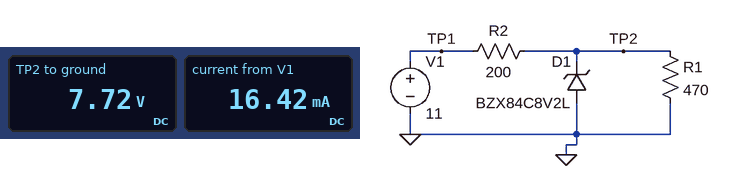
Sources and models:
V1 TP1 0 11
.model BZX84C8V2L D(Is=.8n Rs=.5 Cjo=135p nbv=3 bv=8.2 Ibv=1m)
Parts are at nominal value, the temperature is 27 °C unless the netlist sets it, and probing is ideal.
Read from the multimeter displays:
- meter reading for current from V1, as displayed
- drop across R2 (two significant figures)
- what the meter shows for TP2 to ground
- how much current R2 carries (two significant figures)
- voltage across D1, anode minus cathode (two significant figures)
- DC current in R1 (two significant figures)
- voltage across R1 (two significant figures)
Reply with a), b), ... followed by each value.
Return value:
a) 16.42 mA
b) 3.3 V
c) 7.72 V
d) 16 mA
e) -7.7 V
f) 16 mA
g) 7.7 V
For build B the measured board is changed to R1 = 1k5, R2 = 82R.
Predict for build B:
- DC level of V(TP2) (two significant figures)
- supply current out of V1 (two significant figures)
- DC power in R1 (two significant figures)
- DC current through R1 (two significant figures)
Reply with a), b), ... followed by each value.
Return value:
a) 8.5 V
b) 31 mA
c) 48 mW
d) 5.6 mA
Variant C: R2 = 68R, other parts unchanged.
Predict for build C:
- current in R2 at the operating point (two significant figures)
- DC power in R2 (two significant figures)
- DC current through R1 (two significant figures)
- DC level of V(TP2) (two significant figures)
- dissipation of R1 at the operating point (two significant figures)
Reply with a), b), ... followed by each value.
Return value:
a) 38 mA
b) 96 mW
c) 18 mA
d) 8.4 V
e) 150 mW
